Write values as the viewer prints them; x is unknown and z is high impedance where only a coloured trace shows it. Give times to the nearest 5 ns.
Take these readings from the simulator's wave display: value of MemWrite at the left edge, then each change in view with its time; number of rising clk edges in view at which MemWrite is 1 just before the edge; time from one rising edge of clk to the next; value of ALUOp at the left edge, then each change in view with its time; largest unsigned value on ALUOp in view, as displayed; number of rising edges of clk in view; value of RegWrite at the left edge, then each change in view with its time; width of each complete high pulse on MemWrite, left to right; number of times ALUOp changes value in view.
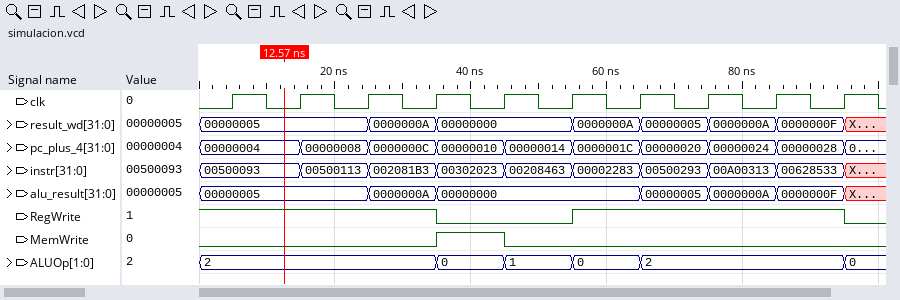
0, 1 at 35 ns, 0 at 45 ns
1
10 ns
2, 0 at 35 ns, 1 at 45 ns, 0 at 55 ns, 2 at 65 ns, 0 at 95 ns
2
10
1, 0 at 35 ns, 1 at 55 ns, 0 at 95 ns
10 ns
5
